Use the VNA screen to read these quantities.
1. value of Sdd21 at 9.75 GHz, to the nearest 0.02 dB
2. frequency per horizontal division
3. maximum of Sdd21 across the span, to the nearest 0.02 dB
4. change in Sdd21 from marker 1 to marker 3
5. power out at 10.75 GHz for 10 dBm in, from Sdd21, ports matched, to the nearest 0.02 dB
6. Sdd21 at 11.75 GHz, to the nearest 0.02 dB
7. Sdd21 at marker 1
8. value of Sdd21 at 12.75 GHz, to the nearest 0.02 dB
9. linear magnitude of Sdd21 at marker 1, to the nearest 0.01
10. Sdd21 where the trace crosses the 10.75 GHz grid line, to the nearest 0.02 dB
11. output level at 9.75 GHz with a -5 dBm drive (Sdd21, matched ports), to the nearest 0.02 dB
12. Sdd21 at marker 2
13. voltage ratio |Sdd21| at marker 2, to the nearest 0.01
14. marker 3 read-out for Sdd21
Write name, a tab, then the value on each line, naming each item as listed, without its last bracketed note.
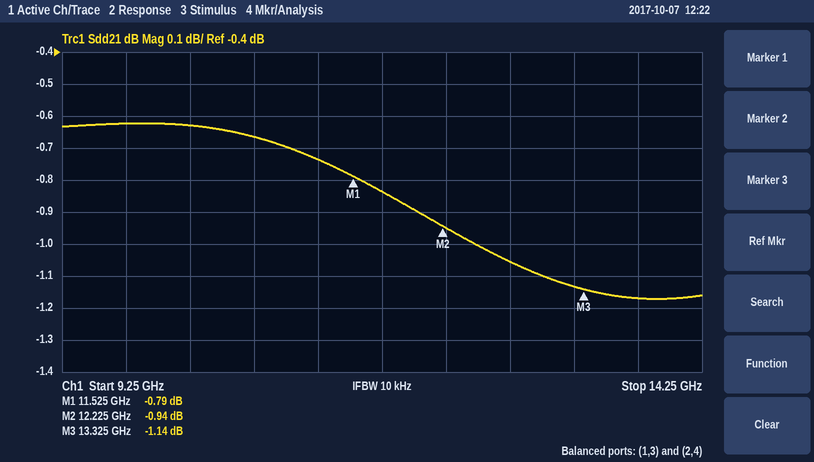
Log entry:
value of Sdd21 at 9.75 GHz, to the nearest 0.02 dB	-0.62 dB
frequency per horizontal division	500 MHz
maximum of Sdd21 across the span, to the nearest 0.02 dB	-0.62 dB
change in Sdd21 from marker 1 to marker 3	-0.35 dB
power out at 10.75 GHz for 10 dBm in, from Sdd21, ports matched, to the nearest 0.02 dB	9.34 dBm
Sdd21 at 11.75 GHz, to the nearest 0.02 dB	-0.84 dB
Sdd21 at marker 1	-0.79 dB
value of Sdd21 at 12.75 GHz, to the nearest 0.02 dB	-1.06 dB
linear magnitude of Sdd21 at marker 1, to the nearest 0.01	0.91
Sdd21 where the trace crosses the 10.75 GHz grid line, to the nearest 0.02 dB	-0.66 dB
output level at 9.75 GHz with a -5 dBm drive (Sdd21, matched ports), to the nearest 0.02 dB	-5.62 dBm
Sdd21 at marker 2	-0.94 dB
voltage ratio |Sdd21| at marker 2, to the nearest 0.01	0.90
marker 3 read-out for Sdd21	-1.14 dB
